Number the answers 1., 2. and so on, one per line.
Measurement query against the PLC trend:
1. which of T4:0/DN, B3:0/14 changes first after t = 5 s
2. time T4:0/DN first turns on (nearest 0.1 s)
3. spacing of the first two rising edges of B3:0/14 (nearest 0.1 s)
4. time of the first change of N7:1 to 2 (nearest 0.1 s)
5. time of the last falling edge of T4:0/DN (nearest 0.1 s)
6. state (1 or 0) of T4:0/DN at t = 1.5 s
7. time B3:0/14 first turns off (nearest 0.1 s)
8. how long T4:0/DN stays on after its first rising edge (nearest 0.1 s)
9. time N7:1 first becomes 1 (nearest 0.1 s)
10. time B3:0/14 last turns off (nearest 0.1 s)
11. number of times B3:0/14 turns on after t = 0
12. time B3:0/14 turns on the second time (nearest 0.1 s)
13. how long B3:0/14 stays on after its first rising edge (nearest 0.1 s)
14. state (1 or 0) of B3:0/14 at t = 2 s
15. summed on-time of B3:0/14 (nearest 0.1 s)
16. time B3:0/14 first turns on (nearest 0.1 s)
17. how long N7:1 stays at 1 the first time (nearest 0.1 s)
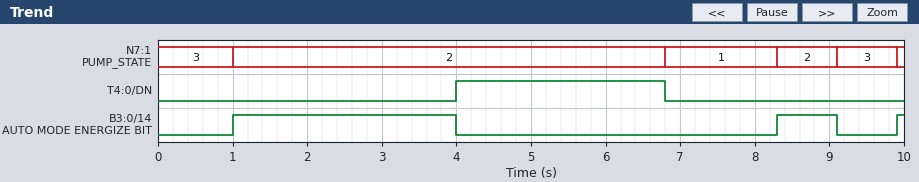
1. T4:0/DN
2. 4.0 s
3. 7.3 s
4. 1.0 s
5. 6.8 s
6. 0
7. 4.0 s
8. 2.8 s
9. 6.8 s
10. 9.1 s
11. 3
12. 8.3 s
13. 3.0 s
14. 1
15. 3.9 s
16. 1.0 s
17. 1.5 s
